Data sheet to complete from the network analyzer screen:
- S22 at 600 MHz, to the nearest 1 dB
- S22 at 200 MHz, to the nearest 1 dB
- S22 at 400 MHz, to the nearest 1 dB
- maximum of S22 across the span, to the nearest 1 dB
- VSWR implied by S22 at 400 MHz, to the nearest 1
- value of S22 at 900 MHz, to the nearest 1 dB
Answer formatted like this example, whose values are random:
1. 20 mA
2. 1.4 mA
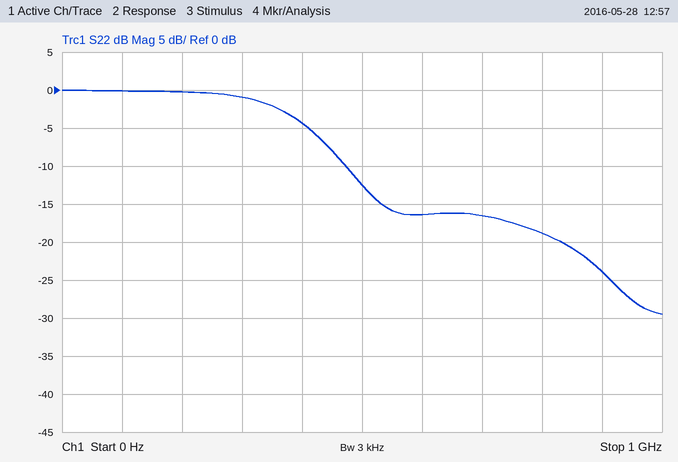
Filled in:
1. -16 dB
2. 0 dB
3. -4 dB
4. 0 dB
5. 4
6. -24 dB
